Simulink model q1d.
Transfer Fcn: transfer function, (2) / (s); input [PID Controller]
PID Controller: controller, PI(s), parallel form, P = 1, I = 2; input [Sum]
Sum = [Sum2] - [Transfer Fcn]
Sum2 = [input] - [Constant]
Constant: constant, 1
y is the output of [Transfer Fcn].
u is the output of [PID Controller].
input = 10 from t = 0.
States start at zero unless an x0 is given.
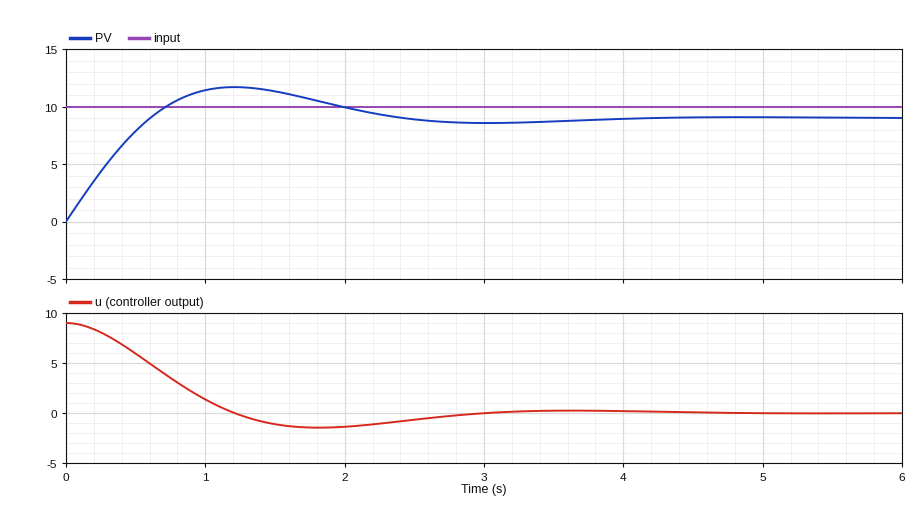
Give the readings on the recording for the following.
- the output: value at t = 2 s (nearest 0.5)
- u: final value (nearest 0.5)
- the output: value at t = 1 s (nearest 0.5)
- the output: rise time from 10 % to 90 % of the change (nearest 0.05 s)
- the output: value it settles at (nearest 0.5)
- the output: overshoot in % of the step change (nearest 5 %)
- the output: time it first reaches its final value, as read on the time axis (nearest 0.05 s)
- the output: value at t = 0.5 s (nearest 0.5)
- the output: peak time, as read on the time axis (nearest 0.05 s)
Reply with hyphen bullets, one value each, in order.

- 10.0
- 0.0
- 11.5
- 0.45 s
- 9.0
- 30 %
- 0.60 s
- 8.0
- 1.20 s
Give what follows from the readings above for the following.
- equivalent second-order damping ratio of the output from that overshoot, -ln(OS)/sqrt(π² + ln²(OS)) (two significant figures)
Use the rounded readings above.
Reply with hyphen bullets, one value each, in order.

- 0.36
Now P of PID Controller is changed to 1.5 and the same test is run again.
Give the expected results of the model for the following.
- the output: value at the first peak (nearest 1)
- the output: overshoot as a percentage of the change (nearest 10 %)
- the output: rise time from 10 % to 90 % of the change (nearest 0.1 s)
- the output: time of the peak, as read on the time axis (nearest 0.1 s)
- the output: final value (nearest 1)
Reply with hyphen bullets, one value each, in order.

- 11
- 20 %
- 0.4 s
- 1.1 s
- 9
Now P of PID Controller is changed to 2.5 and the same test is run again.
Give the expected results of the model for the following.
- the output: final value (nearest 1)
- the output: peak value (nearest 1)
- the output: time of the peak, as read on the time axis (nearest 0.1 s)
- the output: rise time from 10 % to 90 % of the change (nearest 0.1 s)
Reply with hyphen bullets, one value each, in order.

- 9
- 10
- 0.9 s
- 0.3 s
